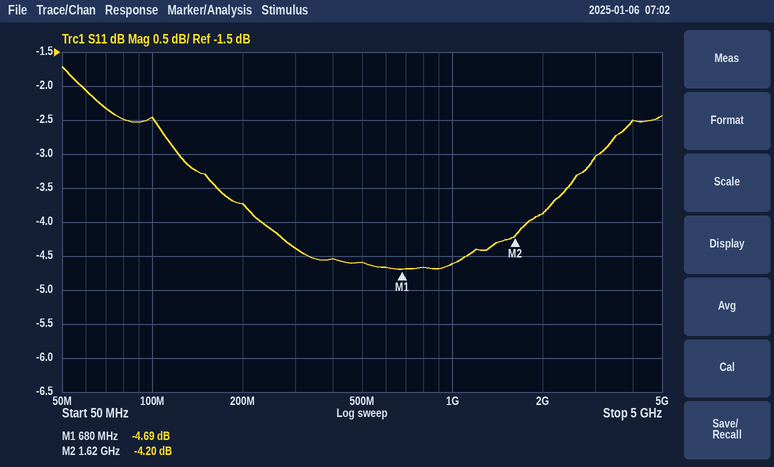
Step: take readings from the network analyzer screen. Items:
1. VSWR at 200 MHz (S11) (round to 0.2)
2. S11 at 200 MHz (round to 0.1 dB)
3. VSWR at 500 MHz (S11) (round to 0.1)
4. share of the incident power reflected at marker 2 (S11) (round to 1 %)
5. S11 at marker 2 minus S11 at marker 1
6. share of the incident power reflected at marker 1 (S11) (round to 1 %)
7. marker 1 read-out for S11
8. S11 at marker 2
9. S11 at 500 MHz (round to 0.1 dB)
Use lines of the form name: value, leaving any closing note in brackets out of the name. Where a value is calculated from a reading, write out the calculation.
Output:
VSWR at 200 MHz (S11): |Γ| = 10^(-3.7/20) = 0.6531; VSWR = (1 + 0.6531)/(1 − 0.6531) ≈ 4.8
S11 at 200 MHz: -3.7 dB
VSWR at 500 MHz (S11): |Γ| = 10^(-4.6/20) = 0.5888; VSWR = (1 + 0.5888)/(1 − 0.5888) ≈ 3.9
share of the incident power reflected at marker 2 (S11): 10^(-4.2/10) ≈ 38 %
S11 at marker 2 minus S11 at marker 1: -4.2 − (-4.69) = 0.49 dB
share of the incident power reflected at marker 1 (S11): 10^(-4.69/10) ≈ 34 %
marker 1 read-out for S11: -4.69 dB
S11 at marker 2: -4.20 dB
S11 at 500 MHz: -4.6 dB
